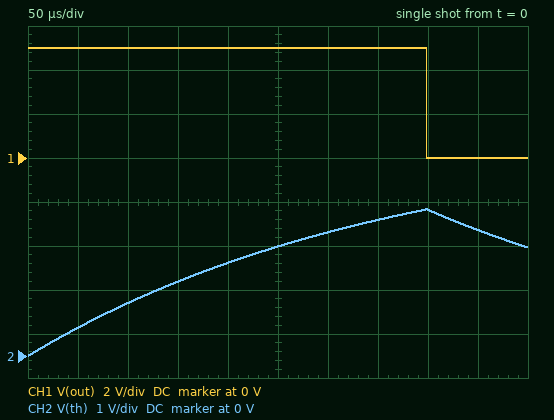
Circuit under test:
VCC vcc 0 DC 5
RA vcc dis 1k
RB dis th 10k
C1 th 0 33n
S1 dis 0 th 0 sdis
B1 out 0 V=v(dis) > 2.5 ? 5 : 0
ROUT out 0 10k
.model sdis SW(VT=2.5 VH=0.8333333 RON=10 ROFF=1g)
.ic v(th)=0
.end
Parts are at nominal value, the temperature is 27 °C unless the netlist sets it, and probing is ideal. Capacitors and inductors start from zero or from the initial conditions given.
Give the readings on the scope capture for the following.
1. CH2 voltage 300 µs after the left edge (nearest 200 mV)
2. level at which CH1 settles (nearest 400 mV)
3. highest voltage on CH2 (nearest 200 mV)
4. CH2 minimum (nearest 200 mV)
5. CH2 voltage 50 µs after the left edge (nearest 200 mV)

2.8 V
0 V
3.4 V
0 V
600 mV
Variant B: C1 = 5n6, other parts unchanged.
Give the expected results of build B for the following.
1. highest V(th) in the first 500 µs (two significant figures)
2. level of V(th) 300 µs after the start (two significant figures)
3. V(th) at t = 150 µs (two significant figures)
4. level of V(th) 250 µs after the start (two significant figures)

3.3 V
2.9 V
3.3 V
2.4 V
